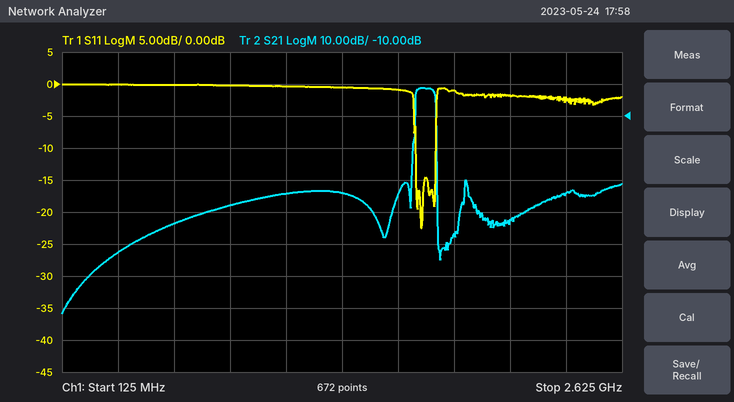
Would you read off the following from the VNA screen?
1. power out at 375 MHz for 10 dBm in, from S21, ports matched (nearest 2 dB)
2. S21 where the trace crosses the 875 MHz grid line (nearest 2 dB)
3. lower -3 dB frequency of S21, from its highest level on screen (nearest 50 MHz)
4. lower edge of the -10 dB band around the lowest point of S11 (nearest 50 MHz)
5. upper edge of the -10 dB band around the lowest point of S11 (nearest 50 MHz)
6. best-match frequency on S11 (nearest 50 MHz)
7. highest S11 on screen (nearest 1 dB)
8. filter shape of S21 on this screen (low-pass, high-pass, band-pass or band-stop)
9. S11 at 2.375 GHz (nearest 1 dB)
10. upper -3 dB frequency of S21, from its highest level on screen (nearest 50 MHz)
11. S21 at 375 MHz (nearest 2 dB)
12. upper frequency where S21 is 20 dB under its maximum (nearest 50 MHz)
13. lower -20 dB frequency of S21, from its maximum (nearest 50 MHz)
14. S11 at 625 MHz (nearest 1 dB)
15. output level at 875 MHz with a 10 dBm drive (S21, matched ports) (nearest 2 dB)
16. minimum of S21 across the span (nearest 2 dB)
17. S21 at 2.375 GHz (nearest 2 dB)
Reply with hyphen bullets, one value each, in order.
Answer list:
- -42 dBm
- -38 dB
- 1.70 GHz
- 1.70 GHz
- 1.80 GHz
- 1.75 GHz
- 0 dB
- band-pass
- -2 dB
- 1.80 GHz
- -52 dB
- 1.80 GHz
- 1.70 GHz
- 0 dB
- -28 dBm
- -72 dB
- -34 dB
